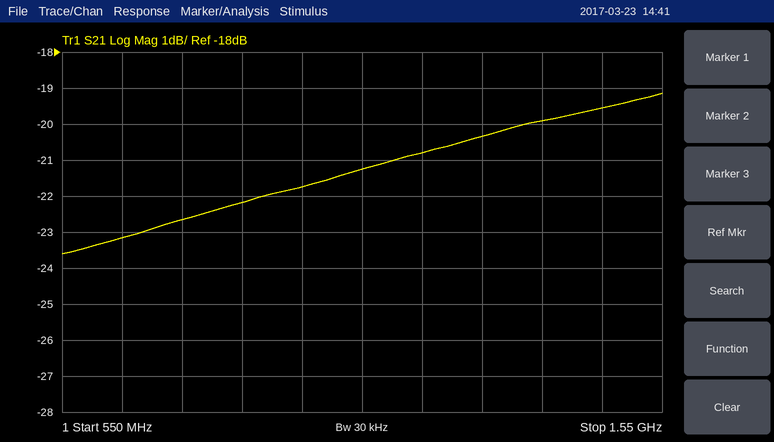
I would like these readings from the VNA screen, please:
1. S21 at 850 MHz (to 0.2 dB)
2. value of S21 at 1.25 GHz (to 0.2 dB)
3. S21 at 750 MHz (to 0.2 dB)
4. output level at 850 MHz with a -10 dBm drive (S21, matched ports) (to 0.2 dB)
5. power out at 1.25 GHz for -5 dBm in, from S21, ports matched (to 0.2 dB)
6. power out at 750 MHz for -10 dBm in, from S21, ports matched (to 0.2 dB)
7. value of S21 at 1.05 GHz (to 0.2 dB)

-22.2 dB
-20.4 dB
-22.6 dB
-32.2 dBm
-25.4 dBm
-32.6 dBm
-21.2 dB
